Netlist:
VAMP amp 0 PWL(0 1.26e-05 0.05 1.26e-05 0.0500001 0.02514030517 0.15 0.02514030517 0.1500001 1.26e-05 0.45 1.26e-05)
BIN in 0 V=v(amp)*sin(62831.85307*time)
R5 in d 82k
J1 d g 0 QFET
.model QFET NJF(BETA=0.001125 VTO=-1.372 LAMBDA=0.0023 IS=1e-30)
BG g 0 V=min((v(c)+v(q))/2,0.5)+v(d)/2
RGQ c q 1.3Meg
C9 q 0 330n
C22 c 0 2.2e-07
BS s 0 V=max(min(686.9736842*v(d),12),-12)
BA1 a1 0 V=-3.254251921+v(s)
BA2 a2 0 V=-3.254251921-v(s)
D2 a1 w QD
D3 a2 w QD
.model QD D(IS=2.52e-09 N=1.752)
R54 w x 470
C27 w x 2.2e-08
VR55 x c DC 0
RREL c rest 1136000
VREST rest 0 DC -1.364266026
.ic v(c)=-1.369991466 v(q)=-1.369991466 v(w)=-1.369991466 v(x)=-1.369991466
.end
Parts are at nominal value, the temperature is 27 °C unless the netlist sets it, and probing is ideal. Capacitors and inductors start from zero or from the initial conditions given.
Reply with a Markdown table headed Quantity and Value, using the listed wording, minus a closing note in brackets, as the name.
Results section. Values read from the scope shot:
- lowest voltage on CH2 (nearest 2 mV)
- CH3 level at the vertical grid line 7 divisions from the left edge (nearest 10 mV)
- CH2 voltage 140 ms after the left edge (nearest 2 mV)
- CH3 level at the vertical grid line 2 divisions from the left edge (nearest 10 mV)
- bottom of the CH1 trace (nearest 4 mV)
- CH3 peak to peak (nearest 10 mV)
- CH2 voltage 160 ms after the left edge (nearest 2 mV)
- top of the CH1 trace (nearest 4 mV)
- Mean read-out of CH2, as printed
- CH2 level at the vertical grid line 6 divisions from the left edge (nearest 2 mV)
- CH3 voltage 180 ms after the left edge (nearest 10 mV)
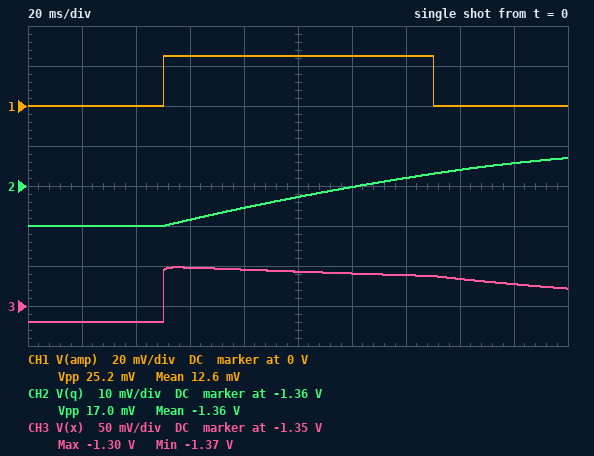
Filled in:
| Quantity | Value |
|---|---|
| lowest voltage on CH2 | -1.370 V |
| CH3 level at the vertical grid line 7 divisions from the left edge | -1.31 V |
| CH2 voltage 140 ms after the left edge | -1.358 V |
| CH3 level at the vertical grid line 2 divisions from the left edge | -1.37 V |
| bottom of the CH1 trace | 0 V |
| CH3 peak to peak | 70 mV |
| CH2 voltage 160 ms after the left edge | -1.356 V |
| top of the CH1 trace | 24 mV |
| Mean read-out of CH2, as printed | -1.36 V |
| CH2 level at the vertical grid line 6 divisions from the left edge | -1.360 V |
| CH3 voltage 180 ms after the left edge | -1.32 V |
